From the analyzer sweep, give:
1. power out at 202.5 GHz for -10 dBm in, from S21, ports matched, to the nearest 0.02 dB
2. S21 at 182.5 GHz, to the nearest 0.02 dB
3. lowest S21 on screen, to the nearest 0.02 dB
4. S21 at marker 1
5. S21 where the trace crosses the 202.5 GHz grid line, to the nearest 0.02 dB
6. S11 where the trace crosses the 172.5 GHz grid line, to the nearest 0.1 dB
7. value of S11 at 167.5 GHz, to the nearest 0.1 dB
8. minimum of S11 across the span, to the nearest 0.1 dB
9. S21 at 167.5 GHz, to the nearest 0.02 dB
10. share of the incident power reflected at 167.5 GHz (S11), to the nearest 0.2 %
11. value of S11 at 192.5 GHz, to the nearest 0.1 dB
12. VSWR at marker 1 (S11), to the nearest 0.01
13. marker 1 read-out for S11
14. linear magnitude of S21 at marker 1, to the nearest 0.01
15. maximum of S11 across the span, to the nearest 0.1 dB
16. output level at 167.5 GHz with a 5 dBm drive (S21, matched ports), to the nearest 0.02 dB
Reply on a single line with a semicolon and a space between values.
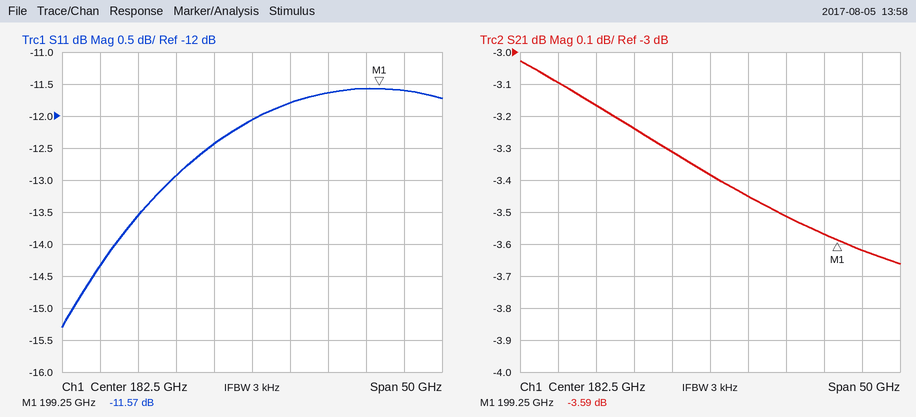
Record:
-13.62 dBm; -3.38 dB; -3.66 dB; -3.59 dB; -3.62 dB; -12.9 dB; -13.6 dB; -15.3 dB; -3.16 dB; 4.4 %; -11.6 dB; 1.72; -11.57 dB; 0.66; -11.6 dB; 1.84 dBm
